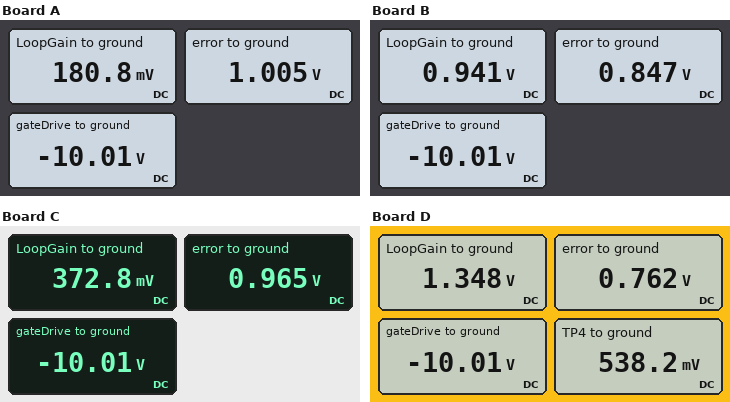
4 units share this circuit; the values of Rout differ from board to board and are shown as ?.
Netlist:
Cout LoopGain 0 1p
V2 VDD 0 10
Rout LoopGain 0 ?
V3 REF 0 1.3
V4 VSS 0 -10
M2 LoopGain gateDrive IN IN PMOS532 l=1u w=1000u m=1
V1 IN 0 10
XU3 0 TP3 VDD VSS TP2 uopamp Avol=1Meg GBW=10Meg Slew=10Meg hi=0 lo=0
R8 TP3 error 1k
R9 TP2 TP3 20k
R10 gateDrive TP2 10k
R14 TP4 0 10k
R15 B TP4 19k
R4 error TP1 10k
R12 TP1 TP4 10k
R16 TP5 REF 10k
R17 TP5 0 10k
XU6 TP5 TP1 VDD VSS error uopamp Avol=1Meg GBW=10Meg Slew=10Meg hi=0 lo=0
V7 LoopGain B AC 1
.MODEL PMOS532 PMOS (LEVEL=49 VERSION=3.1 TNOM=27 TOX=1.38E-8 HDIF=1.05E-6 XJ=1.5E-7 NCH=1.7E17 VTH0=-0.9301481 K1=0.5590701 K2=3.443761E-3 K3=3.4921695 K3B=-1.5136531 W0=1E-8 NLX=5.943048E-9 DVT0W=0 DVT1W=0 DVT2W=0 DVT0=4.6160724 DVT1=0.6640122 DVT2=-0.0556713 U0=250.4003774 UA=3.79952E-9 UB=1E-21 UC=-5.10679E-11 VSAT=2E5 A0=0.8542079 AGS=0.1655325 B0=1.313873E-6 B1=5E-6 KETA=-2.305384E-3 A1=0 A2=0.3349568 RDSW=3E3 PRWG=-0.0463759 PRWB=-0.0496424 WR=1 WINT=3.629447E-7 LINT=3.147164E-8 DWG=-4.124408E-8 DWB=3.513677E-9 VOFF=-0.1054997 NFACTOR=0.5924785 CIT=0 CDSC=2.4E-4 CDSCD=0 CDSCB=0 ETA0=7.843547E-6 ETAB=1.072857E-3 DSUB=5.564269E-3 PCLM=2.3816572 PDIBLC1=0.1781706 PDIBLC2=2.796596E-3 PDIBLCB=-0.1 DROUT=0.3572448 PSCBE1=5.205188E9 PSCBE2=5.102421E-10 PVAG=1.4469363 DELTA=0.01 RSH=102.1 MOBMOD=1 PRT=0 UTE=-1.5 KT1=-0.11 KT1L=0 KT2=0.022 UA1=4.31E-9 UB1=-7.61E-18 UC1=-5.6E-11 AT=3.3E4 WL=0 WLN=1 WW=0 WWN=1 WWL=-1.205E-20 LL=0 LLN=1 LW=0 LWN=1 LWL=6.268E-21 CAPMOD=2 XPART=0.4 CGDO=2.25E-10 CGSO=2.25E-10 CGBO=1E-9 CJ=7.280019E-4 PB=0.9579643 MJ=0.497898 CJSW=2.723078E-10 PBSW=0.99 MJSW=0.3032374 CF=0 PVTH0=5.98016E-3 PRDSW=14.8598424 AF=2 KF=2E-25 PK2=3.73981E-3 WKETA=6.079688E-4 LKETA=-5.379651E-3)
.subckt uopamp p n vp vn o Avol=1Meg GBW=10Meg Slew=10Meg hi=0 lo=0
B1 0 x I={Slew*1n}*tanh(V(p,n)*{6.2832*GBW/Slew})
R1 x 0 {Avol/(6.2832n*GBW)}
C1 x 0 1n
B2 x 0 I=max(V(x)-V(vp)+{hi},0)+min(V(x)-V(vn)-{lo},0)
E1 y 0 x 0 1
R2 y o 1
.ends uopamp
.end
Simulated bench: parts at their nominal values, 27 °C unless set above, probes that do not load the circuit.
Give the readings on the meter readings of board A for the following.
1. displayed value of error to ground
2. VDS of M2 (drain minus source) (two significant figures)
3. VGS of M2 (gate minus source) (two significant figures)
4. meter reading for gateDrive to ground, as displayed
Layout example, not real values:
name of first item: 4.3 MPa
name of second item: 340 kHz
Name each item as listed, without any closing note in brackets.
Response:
displayed value of error to ground: 1.005 V
VDS of M2 (drain minus source): -9.8 V
VGS of M2 (gate minus source): -20 V
meter reading for gateDrive to ground, as displayed: -10.01 V
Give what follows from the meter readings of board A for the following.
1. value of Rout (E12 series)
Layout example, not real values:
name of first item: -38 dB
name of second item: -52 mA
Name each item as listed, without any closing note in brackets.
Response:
value of Rout: 3.9 Ω
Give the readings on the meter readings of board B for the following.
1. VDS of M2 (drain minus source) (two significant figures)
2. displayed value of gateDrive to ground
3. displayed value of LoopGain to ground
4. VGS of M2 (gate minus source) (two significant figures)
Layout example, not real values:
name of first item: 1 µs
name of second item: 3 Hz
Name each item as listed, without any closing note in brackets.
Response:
VDS of M2 (drain minus source): -9.1 V
displayed value of gateDrive to ground: -10.01 V
displayed value of LoopGain to ground: 0.941 V
VGS of M2 (gate minus source): -20 V
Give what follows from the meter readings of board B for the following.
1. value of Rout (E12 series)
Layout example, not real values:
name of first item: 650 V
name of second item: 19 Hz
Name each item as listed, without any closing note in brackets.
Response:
value of Rout: 22 Ω
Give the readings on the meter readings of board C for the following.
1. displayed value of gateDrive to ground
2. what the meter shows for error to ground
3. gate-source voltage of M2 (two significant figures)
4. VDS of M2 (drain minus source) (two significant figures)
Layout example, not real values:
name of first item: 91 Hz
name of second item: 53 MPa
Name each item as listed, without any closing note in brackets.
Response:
displayed value of gateDrive to ground: -10.01 V
what the meter shows for error to ground: 0.965 V
gate-source voltage of M2: -20 V
VDS of M2 (drain minus source): -9.6 V
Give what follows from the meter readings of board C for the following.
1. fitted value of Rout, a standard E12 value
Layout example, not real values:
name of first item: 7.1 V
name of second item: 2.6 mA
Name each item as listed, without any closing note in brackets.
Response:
fitted value of Rout, a standard E12 value: 8.2 Ω
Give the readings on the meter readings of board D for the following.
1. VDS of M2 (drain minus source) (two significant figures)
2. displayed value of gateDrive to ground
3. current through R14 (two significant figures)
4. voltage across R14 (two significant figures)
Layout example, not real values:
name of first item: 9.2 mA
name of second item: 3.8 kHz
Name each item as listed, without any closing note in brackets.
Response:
VDS of M2 (drain minus source): -8.7 V
displayed value of gateDrive to ground: -10.01 V
current through R14: 54 µA
voltage across R14: 540 mV
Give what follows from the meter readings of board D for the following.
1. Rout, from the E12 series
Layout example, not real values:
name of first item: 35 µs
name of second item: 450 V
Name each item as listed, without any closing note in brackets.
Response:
Rout, from the E12 series: 33 Ω
